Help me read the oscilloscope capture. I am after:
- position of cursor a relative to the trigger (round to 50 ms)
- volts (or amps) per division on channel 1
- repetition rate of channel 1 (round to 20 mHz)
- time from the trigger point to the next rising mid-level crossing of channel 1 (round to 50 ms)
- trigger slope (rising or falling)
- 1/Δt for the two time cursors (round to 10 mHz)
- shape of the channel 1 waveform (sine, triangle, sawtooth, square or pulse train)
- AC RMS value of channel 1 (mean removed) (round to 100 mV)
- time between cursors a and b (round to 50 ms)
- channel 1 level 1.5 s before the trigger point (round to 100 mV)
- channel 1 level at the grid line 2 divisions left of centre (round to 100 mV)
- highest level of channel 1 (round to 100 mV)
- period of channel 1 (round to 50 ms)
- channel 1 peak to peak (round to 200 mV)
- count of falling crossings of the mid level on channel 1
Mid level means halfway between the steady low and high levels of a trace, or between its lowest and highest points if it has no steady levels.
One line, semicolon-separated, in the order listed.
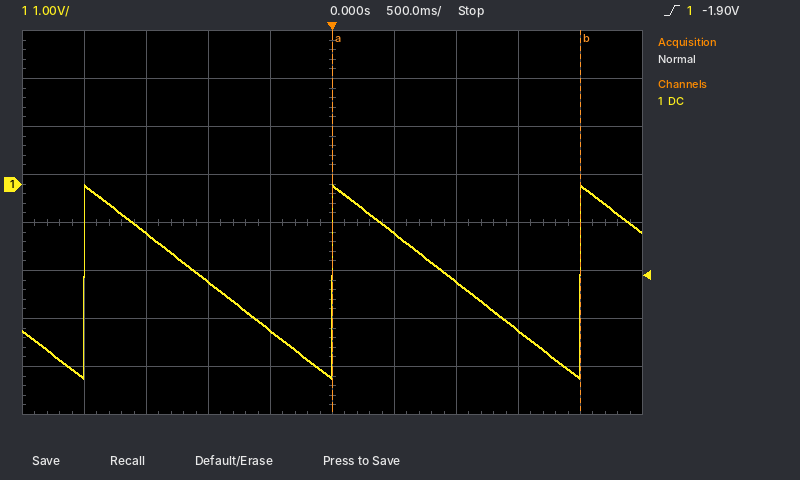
0 ms; 1 V; 500 mHz; 2.00 s; rising; 500 mHz; sawtooth; 1.2 V; 2.00 s; -1.0 V; -2.0 V; 0.0 V; 2.00 s; 4.0 V; 2
